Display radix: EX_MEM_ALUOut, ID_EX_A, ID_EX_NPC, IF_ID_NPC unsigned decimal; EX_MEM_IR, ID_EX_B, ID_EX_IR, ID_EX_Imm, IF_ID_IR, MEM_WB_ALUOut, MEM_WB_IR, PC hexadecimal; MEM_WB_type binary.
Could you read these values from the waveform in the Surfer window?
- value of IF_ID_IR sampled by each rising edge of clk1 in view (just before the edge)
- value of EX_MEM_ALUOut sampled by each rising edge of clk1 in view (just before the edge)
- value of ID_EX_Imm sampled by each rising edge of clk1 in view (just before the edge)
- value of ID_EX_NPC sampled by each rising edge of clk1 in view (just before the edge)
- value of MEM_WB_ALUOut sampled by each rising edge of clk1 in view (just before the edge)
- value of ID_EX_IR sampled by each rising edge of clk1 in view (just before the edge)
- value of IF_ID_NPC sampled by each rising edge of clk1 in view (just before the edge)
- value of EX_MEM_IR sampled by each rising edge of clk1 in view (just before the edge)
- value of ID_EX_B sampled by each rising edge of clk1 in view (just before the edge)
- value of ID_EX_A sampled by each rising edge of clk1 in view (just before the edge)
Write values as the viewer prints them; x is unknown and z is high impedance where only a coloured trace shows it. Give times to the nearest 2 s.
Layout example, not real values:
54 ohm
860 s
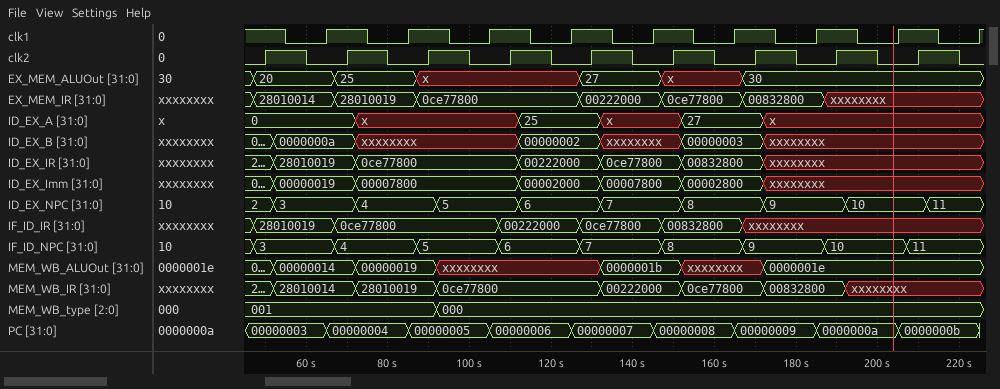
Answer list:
28010019, 0ce77800, 0ce77800, 00222000, 0ce77800, 00832800, xxxxxxxx, xxxxxxxx, xxxxxxxx
20, 25, x, x, 27, x, 30, 30, 30
00000019, 00007800, 00007800, 00002000, 00007800, 00002800, xxxxxxxx, xxxxxxxx, xxxxxxxx
3, 4, 5, 6, 7, 8, 9, 10, 11
00000014, 00000019, xxxxxxxx, xxxxxxxx, 0000001b, xxxxxxxx, 0000001e, 0000001e, 0000001e
28010019, 0ce77800, 0ce77800, 00222000, 0ce77800, 00832800, xxxxxxxx, xxxxxxxx, xxxxxxxx
3, 4, 5, 6, 7, 8, 9, 10, 11
28010014, 28010019, 0ce77800, 0ce77800, 00222000, 0ce77800, 00832800, xxxxxxxx, xxxxxxxx
0000000a, xxxxxxxx, xxxxxxxx, 00000002, xxxxxxxx, 00000003, xxxxxxxx, xxxxxxxx, xxxxxxxx
0, x, x, 25, x, 27, x, x, x
